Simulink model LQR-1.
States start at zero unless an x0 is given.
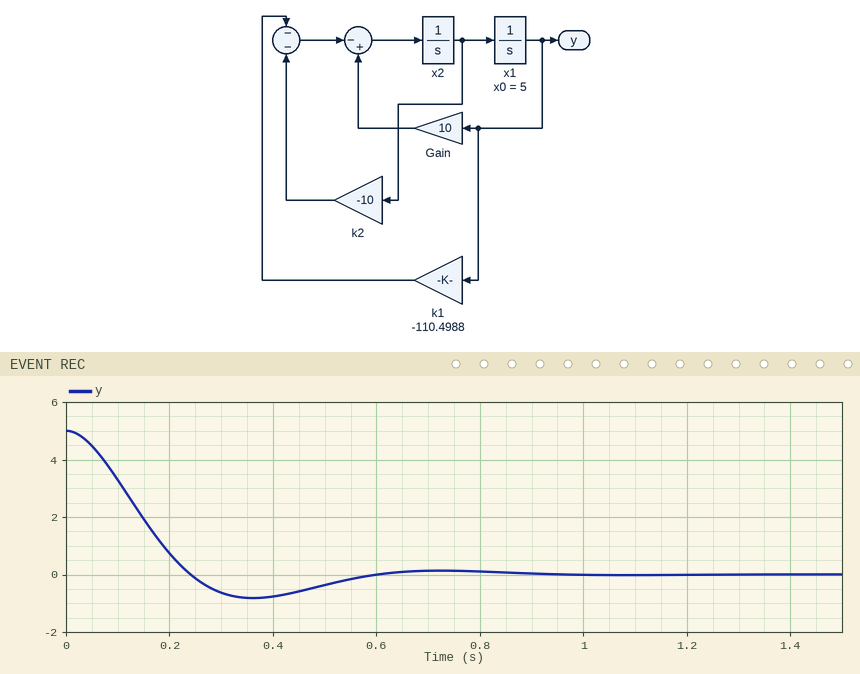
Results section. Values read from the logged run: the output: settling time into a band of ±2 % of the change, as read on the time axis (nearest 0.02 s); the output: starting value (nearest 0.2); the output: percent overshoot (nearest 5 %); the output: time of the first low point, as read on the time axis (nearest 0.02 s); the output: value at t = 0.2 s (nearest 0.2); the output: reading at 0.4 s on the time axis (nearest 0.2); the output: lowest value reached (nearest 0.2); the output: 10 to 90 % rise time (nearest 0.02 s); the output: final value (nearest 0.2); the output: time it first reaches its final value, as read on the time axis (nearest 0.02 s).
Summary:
0.80 s
5.0
15 %
0.36 s
0.8
-0.8
-0.8
0.16 s
0.0
0.24 s
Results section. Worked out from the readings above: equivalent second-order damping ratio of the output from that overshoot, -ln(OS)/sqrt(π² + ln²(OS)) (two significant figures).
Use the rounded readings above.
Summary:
0.52
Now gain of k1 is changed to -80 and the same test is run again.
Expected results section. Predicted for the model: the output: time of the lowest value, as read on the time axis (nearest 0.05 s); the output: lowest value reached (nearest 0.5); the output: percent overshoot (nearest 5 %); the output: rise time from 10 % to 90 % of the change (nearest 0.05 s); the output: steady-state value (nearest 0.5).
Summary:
0.45 s
-0.5
10 %
0.20 s
0.0
